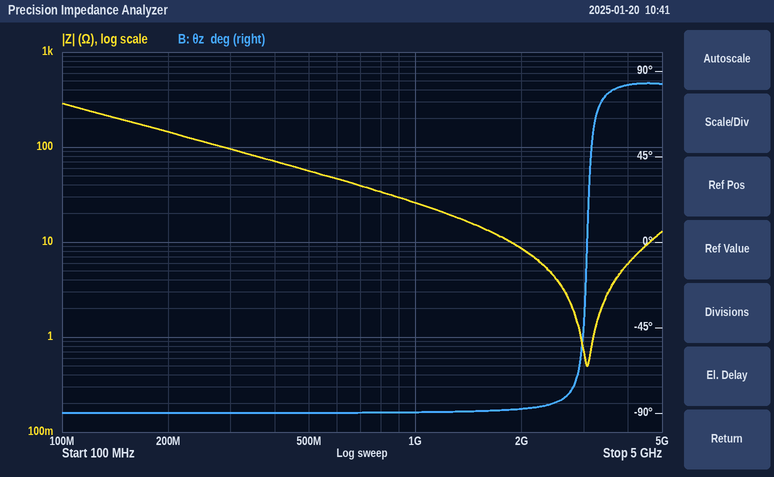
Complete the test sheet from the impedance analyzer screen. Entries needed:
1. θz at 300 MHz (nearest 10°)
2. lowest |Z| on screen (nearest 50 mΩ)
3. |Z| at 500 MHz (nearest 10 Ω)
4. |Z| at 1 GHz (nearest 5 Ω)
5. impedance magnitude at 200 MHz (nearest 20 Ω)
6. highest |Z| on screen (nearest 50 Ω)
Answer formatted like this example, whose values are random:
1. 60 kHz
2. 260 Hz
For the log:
1. -90°
2. 500 mΩ
3. 60 Ω
4. 25 Ω
5. 140 Ω
6. 300 Ω
